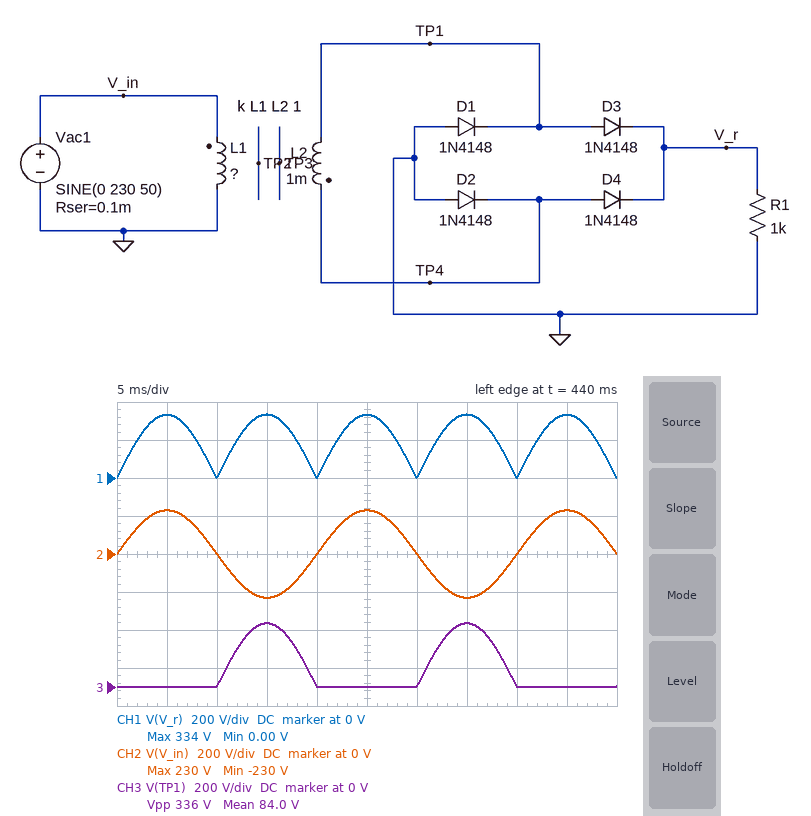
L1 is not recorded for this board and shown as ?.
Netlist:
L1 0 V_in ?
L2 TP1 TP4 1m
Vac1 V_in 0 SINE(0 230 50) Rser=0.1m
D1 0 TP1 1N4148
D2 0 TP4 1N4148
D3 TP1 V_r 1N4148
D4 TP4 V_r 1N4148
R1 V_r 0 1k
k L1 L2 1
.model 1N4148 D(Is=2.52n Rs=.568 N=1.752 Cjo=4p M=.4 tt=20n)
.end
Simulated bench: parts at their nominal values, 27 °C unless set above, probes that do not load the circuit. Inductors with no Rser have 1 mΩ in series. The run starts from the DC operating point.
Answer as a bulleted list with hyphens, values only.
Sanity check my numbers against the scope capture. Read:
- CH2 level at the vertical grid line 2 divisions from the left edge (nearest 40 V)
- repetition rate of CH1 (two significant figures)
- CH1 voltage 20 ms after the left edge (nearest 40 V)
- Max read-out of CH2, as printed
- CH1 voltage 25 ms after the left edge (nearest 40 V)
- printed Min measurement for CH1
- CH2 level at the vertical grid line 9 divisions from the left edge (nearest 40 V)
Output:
- 0 V
- 100 Hz
- 0 V
- 230 V
- 320 V
- 0.00 V
- 240 V
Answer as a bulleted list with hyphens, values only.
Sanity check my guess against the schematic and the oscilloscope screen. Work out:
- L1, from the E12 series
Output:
- 470 µH
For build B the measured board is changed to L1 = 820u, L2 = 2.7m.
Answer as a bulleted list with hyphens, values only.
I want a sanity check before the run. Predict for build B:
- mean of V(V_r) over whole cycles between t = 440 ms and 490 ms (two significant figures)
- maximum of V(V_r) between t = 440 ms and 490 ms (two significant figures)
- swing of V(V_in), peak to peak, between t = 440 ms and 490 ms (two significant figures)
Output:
- 260 V
- 420 V
- 460 V
